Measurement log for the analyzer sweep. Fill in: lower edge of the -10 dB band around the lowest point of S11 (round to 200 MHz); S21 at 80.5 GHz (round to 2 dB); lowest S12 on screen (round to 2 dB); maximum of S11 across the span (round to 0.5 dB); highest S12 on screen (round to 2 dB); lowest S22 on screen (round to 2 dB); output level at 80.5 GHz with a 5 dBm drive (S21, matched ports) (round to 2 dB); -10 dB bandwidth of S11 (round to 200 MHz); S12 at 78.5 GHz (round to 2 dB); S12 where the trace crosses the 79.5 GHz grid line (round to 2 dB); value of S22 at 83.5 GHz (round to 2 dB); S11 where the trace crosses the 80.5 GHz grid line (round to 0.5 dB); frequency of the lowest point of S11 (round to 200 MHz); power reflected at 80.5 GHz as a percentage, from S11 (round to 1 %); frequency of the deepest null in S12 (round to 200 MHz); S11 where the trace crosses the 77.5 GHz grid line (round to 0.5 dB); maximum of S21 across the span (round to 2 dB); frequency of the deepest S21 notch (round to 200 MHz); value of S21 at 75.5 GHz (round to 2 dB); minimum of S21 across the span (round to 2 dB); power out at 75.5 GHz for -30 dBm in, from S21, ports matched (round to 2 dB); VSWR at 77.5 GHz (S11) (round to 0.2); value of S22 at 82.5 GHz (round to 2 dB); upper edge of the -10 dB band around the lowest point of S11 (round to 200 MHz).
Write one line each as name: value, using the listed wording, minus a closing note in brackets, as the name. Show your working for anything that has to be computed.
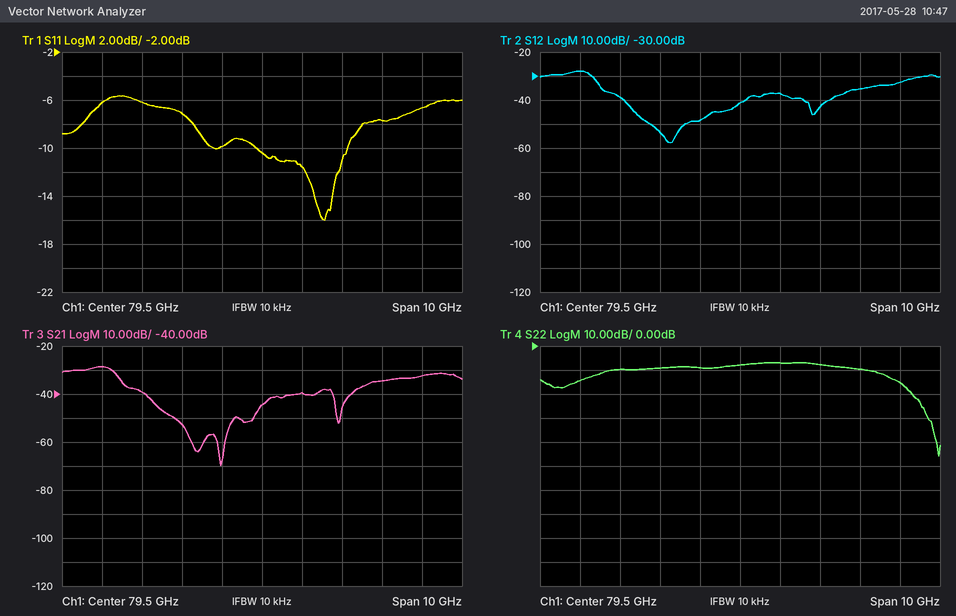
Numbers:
lower edge of the -10 dB band around the lowest point of S11: 79.4 GHz
S21 at 80.5 GHz: -40 dB
lowest S12 on screen: -58 dB
maximum of S11 across the span: -5.5 dB
highest S12 on screen: -28 dB
lowest S22 on screen: -46 dB
output level at 80.5 GHz with a 5 dBm drive (S21, matched ports): 5 dBm + (-40 dB) = -34 dBm
-10 dB bandwidth of S11: 81.6 GHz − 79.4 GHz = 2.2 GHz
S12 at 78.5 GHz: -48 dB
S12 where the trace crosses the 79.5 GHz grid line: -42 dB
value of S22 at 83.5 GHz: -16 dB
S11 where the trace crosses the 80.5 GHz grid line: -11.5 dB
frequency of the lowest point of S11: 81.0 GHz
power reflected at 80.5 GHz as a percentage, from S11: 10^(-11.5/10) ≈ 7 %
frequency of the deepest null in S12: 77.8 GHz
S11 where the trace crosses the 77.5 GHz grid line: -7.0 dB
maximum of S21 across the span: -28 dB
frequency of the deepest S21 notch: 78.4 GHz
value of S21 at 75.5 GHz: -28 dB
minimum of S21 across the span: -70 dB
power out at 75.5 GHz for -30 dBm in, from S21, ports matched: -30 dBm + (-28 dB) = -58 dBm
VSWR at 77.5 GHz (S11): |Γ| = 10^(-7/20) = 0.4467; VSWR = (1 + 0.4467)/(1 − 0.4467) ≈ 2.6
value of S22 at 82.5 GHz: -10 dB
upper edge of the -10 dB band around the lowest point of S11: 81.6 GHz
